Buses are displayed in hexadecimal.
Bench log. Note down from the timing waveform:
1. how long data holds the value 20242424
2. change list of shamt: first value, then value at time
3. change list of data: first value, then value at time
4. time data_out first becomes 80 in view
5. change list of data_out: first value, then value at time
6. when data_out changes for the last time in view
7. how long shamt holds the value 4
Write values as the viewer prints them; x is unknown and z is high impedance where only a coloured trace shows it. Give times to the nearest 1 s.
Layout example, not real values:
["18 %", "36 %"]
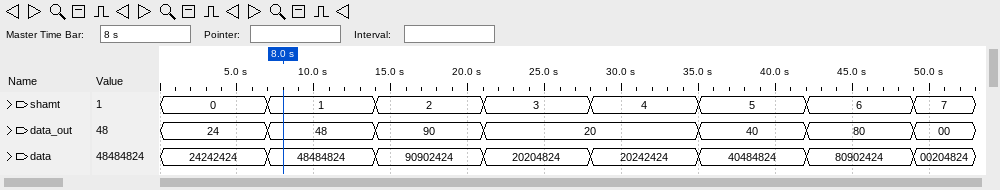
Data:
["7 s", "0, 1 at 7 s, 2 at 14 s, 3 at 21 s, 4 at 28 s, 5 at 35 s, 6 at 42 s, 7 at 49 s", "24242424, 48484824 at 7 s, 90902424 at 14 s, 20204824 at 21 s, 20242424 at 28 s, 40484824 at 35 s, 80902424 at 42 s, 00204824 at 49 s", "42 s", "24, 48 at 7 s, 90 at 14 s, 20 at 21 s, 40 at 35 s, 80 at 42 s, 00 at 49 s", "49 s", "7 s"]
